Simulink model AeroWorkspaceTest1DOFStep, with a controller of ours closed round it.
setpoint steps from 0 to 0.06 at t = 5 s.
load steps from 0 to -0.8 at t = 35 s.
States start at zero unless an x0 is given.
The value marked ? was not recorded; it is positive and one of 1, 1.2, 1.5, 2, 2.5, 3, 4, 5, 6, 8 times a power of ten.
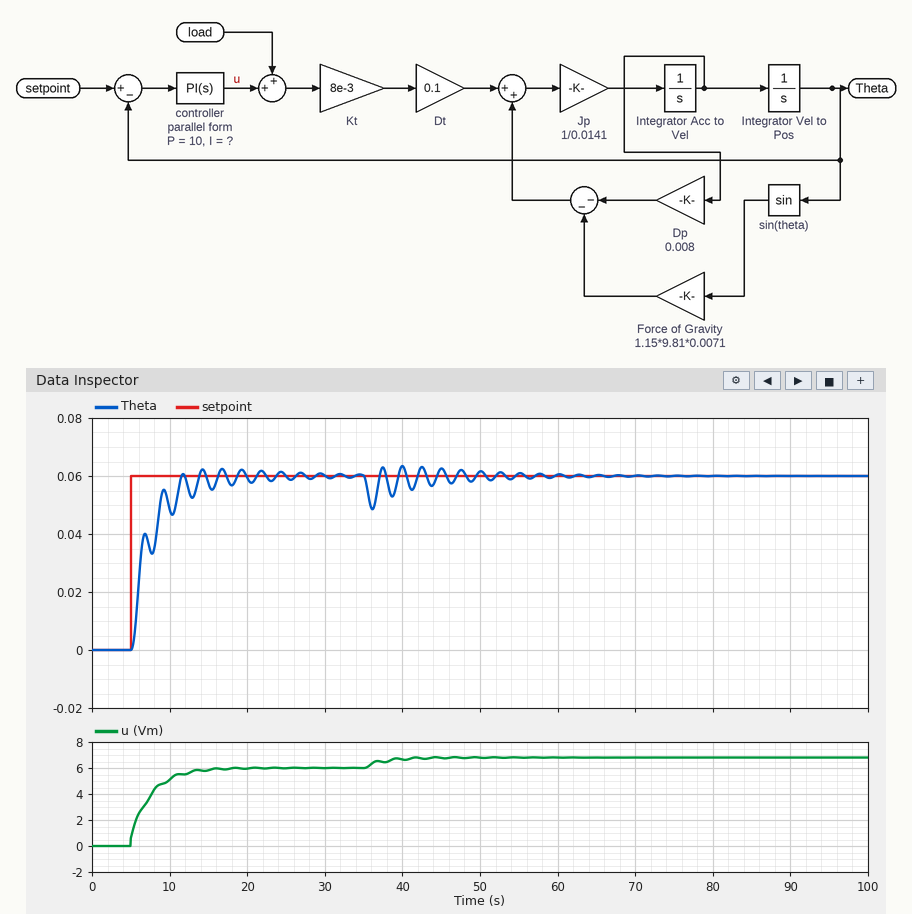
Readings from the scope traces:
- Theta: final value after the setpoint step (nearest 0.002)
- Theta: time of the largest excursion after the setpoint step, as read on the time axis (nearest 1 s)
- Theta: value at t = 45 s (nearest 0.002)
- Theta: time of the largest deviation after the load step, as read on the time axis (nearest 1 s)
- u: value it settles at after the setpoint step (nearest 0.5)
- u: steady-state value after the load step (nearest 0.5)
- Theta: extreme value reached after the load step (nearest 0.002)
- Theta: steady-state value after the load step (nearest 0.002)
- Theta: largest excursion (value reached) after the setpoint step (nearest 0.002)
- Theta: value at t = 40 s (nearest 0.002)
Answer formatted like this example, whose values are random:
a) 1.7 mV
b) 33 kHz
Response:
a) 0.060
b) 17 s
c) 0.062
d) 36 s
e) 6.0
f) 7.0
g) 0.048
h) 0.060
i) 0.062
j) 0.064
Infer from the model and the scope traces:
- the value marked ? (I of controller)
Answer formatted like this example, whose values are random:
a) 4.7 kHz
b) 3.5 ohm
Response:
a) 40
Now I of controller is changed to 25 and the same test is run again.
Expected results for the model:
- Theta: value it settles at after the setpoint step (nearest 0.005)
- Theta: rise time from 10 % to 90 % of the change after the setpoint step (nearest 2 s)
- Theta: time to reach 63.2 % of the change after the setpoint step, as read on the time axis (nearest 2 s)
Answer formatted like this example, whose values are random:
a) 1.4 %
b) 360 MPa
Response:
a) 0.060
b) 8 s
c) 8 s
